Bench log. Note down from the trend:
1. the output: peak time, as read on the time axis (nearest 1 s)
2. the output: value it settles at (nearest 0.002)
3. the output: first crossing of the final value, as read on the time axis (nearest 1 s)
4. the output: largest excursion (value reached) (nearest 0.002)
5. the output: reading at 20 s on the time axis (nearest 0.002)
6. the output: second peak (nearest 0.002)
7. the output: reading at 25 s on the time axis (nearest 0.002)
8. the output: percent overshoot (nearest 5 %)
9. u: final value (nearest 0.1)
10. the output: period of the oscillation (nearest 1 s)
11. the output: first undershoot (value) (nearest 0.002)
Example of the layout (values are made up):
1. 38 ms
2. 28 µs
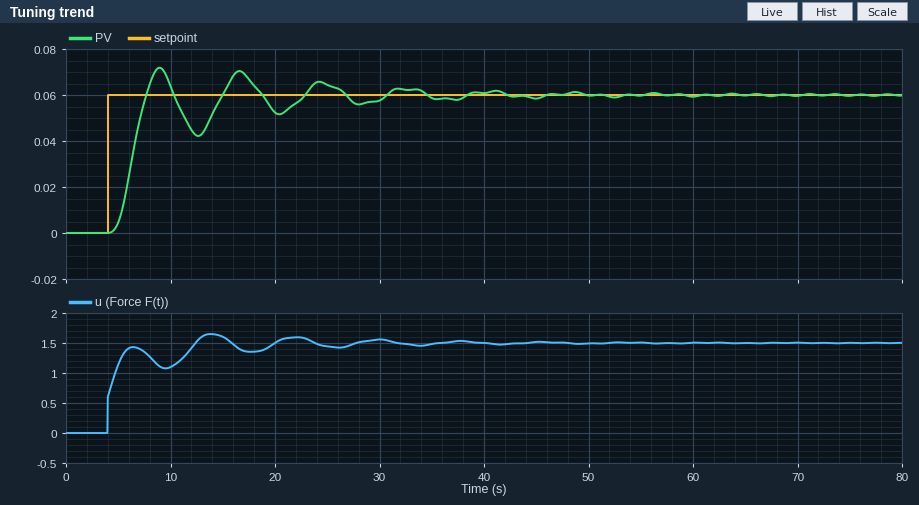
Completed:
1. 9 s
2. 0.060
3. 8 s
4. 0.072
5. 0.052
6. 0.070
7. 0.064
8. 20 %
9. 1.5
10. 8 s
11. 0.042
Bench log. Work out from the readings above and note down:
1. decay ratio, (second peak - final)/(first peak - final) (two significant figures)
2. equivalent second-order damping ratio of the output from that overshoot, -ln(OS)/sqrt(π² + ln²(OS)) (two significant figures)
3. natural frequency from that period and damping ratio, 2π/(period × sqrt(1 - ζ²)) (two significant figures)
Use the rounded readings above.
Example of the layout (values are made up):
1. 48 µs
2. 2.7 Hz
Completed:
1. 0.83
2. 0.46
3. 0.88 rad/s
